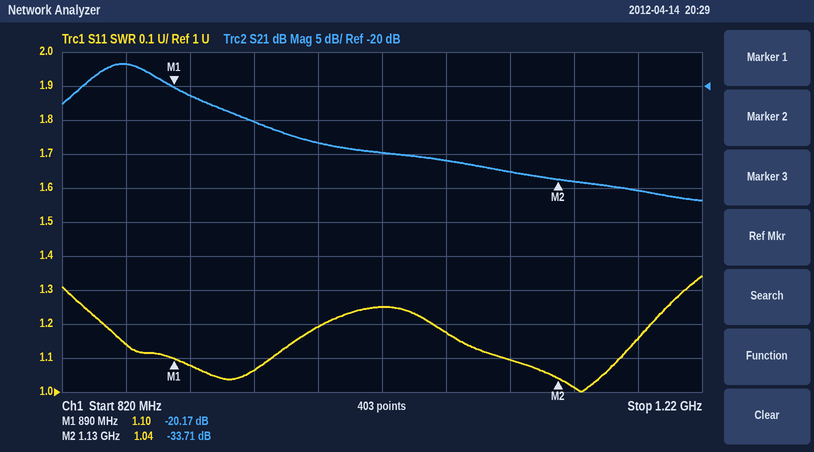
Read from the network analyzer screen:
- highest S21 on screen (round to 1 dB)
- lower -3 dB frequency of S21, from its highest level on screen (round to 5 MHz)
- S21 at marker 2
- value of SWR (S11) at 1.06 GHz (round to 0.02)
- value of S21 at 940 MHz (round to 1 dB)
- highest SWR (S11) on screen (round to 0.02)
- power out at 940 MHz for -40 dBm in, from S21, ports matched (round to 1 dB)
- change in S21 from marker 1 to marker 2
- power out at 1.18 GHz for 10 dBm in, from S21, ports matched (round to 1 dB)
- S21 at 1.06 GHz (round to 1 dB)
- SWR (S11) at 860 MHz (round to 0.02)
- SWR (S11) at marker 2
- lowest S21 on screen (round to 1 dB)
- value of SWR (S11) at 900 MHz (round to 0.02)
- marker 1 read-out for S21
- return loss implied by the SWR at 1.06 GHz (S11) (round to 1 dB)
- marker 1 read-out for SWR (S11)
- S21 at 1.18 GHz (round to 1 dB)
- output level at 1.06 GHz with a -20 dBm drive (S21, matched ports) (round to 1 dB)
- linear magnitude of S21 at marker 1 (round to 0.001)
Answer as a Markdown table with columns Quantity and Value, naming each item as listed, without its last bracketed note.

| Quantity | Value |
|---|---|
| highest S21 on screen | -17 dB |
| lower -3 dB frequency of S21, from its highest level on screen | 835 MHz |
| S21 at marker 2 | -33.71 dB |
| value of SWR (S11) at 1.06 GHz | 1.18 |
| value of S21 at 940 MHz | -25 dB |
| highest SWR (S11) on screen | 1.34 |
| power out at 940 MHz for -40 dBm in, from S21, ports matched | -65 dBm |
| change in S21 from marker 1 to marker 2 | -13.54 dB |
| power out at 1.18 GHz for 10 dBm in, from S21, ports matched | -25 dBm |
| S21 at 1.06 GHz | -31 dB |
| SWR (S11) at 860 MHz | 1.14 |
| SWR (S11) at marker 2 | 1.04 |
| lowest S21 on screen | -37 dB |
| value of SWR (S11) at 900 MHz | 1.08 |
| marker 1 read-out for S21 | -20.17 dB |
| return loss implied by the SWR at 1.06 GHz (S11) | 22 dB |
| marker 1 read-out for SWR | 1.10 |
| S21 at 1.18 GHz | -35 dB |
| output level at 1.06 GHz with a -20 dBm drive (S21, matched ports) | -51 dBm |
| linear magnitude of S21 at marker 1 | 0.098 |
